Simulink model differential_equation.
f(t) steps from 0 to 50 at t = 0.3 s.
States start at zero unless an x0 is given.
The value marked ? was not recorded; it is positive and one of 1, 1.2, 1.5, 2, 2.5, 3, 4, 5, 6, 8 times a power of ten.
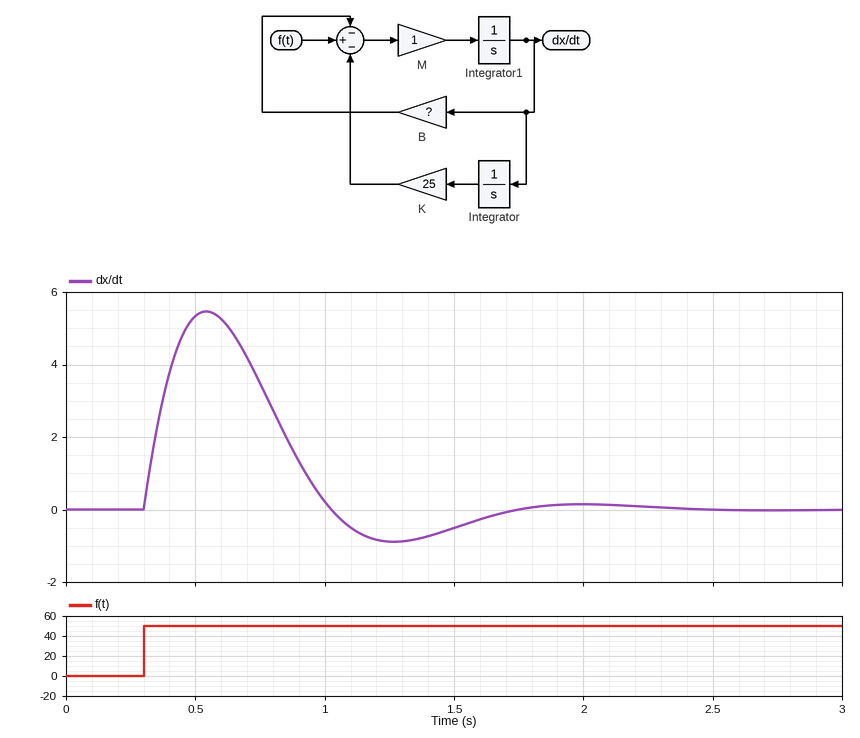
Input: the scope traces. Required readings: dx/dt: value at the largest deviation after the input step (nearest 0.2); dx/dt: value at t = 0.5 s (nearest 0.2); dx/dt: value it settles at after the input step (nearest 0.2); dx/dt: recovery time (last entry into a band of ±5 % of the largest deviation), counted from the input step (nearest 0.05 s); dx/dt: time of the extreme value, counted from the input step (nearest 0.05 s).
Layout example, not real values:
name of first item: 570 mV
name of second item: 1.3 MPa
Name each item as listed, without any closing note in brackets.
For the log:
dx/dt: value at the largest deviation after the input step: 5.4
dx/dt: value at t = 0.5 s: 5.4
dx/dt: value it settles at after the input step: 0.0
dx/dt: recovery time (last entry into a band of ±5 % of the largest deviation), counted from the input step: 1.30 s
dx/dt: time of the extreme value, counted from the input step: 0.25 s
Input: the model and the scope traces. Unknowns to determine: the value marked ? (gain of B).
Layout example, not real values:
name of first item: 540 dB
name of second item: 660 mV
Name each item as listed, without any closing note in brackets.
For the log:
the value marked ?: 5
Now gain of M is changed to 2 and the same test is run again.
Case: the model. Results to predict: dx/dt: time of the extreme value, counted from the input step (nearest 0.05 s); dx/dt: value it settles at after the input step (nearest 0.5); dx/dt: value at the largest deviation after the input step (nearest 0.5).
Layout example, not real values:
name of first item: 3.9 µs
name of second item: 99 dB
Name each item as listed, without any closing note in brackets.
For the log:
dx/dt: time of the extreme value, counted from the input step: 0.15 s
dx/dt: value it settles at after the input step: 0.0
dx/dt: value at the largest deviation after the input step: 6.5
